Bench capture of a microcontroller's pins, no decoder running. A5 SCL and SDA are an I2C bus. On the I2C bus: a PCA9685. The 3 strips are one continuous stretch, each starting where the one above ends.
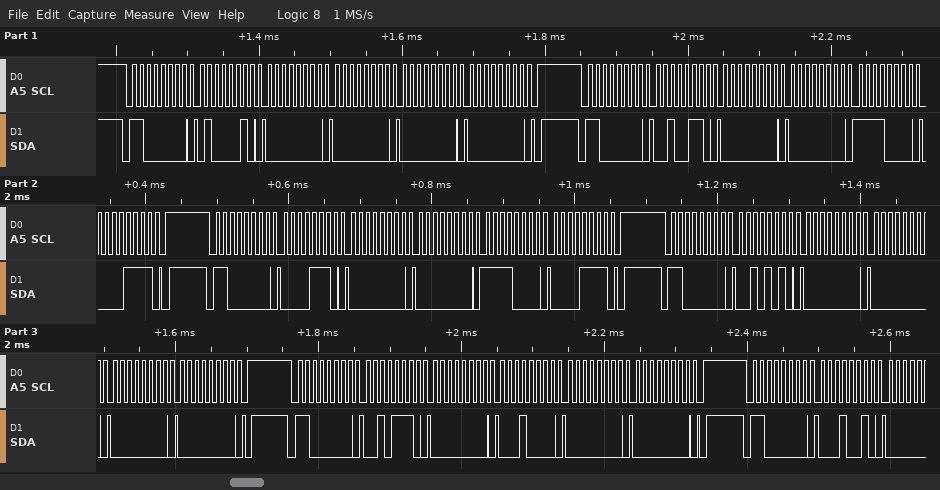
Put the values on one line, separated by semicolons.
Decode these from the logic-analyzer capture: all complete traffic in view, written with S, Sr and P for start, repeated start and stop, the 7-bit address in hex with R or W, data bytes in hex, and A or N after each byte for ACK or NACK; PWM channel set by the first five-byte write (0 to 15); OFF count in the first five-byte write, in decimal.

S 60W A 42 A 00 A 00 A 00 A 00 A P S 60W A 26 A 00 A 00 A F0 A 0F A P S 60W A 0E A 00 A 00 A F0 A 0F A P S 60W A 2A A 00 A 00 A 00 A 00 A P S 60W A 2E A 00 A 10 A 00 A 00 A P S 60W A 12 A; 15; 0
